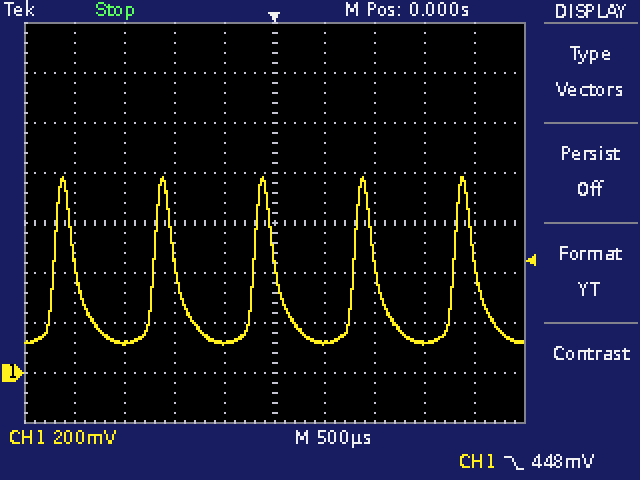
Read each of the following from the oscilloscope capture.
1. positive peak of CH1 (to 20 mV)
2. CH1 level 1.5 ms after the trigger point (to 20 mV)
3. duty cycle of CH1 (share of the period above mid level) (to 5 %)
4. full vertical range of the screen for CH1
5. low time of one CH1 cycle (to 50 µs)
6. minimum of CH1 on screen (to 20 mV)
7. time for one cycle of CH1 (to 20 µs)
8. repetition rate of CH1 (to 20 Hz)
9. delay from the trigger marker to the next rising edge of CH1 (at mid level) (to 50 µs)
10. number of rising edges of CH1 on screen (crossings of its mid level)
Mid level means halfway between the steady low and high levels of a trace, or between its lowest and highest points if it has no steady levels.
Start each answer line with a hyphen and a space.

- 780 mV
- 120 mV
- 20 %
- 1.6 V
- 800 µs
- 120 mV
- 1.00 ms
- 1.00 kHz
- 800 µs
- 5
